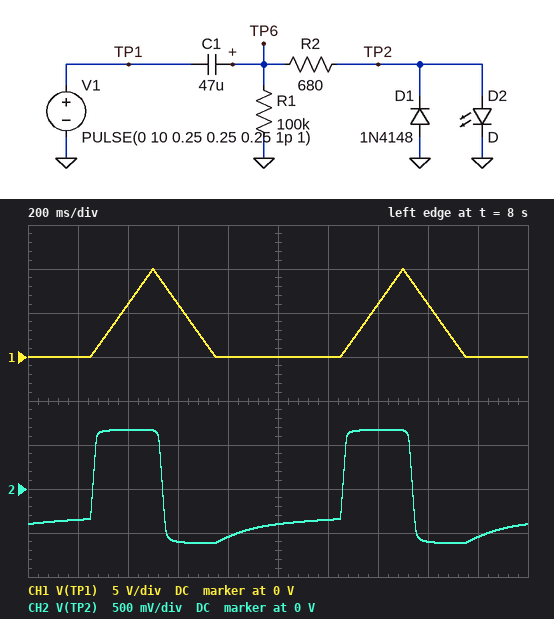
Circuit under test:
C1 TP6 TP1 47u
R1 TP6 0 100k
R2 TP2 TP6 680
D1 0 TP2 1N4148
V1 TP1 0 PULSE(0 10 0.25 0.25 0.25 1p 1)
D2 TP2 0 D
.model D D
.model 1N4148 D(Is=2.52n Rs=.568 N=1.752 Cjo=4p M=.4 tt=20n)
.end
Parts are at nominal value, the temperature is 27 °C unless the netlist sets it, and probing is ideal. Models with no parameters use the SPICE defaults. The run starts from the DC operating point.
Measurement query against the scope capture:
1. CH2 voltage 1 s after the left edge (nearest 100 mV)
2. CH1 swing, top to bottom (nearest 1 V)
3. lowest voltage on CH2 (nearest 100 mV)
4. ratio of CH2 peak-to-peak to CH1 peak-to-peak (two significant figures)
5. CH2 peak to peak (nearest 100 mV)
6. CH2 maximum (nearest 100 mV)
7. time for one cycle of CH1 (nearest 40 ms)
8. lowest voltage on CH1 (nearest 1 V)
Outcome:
-400 mV
10 V
-600 mV
0.13
1.3 V
700 mV
1.00 s
0 V
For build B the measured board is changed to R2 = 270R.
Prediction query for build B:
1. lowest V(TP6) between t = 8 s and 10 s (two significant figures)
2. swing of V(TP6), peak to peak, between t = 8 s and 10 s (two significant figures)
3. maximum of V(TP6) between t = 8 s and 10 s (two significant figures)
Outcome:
-1.1 V
2.3 V
1.2 V
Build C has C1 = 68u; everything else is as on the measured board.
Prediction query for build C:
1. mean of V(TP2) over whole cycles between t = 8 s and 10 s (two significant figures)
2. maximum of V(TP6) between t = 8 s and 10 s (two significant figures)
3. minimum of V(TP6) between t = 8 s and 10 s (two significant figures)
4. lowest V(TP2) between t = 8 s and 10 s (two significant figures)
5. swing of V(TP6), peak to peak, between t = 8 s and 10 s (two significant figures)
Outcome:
-170 mV
2.5 V
-2.4 V
-630 mV
4.9 V
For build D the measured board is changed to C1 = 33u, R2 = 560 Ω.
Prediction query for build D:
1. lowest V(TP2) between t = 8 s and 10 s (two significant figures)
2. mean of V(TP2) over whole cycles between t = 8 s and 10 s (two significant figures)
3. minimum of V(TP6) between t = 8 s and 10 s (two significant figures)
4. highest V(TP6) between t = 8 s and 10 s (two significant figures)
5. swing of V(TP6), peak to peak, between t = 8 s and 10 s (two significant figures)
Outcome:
-600 mV
-150 mV
-1.3 V
1.4 V
2.7 V
